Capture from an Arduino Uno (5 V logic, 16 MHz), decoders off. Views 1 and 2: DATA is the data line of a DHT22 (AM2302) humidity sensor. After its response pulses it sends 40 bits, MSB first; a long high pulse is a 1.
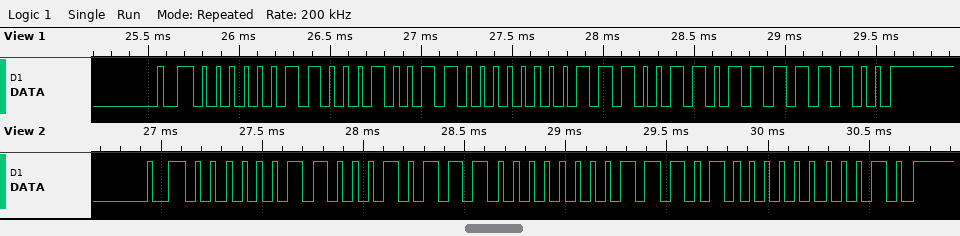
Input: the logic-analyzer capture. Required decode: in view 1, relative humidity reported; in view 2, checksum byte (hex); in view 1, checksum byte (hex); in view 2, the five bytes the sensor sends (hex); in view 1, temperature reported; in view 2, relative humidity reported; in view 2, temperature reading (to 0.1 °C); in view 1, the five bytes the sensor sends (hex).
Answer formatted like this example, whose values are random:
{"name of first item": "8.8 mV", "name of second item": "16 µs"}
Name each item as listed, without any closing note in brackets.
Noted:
{"in view 1, relative humidity reported": "78.7 %", "in view 2, checksum byte": "0x02", "in view 1, checksum byte": "0xFC", "in view 2, the five bytes the sensor sends": "03 17 00 E8 02", "in view 1, temperature reported": "23.0 °C", "in view 2, relative humidity reported": "79.1 %", "in view 2, temperature reading": "23.2 °C", "in view 1, the five bytes the sensor sends": "03 13 00 E6 FC"}
